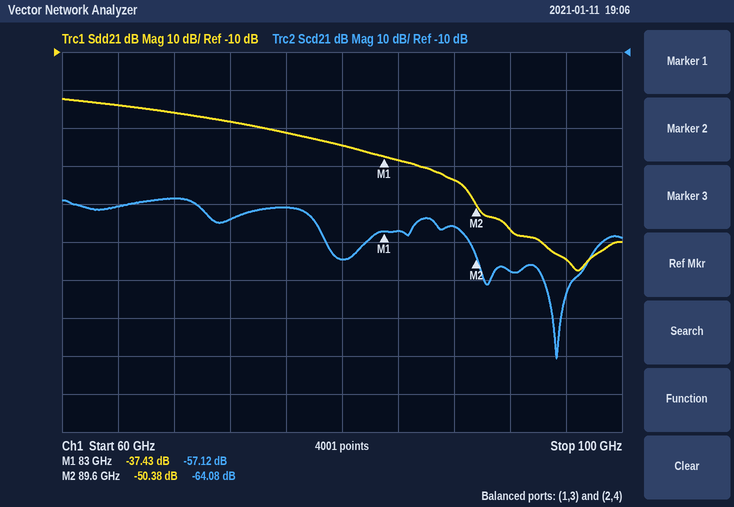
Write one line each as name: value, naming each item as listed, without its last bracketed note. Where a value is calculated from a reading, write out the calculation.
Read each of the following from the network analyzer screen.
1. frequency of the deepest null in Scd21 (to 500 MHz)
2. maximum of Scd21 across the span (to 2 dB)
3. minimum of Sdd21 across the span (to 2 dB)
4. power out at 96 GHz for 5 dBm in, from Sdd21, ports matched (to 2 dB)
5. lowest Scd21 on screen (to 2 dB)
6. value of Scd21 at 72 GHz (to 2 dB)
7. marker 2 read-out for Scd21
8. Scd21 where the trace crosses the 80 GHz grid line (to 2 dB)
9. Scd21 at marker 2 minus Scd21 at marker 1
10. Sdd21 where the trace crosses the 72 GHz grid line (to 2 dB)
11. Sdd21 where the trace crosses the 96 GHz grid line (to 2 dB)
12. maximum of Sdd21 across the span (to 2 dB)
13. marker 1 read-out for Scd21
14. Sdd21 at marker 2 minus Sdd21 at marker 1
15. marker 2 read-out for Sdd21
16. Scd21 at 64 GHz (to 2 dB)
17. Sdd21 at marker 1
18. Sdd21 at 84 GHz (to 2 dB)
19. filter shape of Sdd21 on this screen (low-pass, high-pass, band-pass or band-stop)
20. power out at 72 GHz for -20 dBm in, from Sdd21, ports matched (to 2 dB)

frequency of the deepest null in Scd21: 95.5 GHz
maximum of Scd21 across the span: -48 dB
minimum of Sdd21 across the span: -68 dB
power out at 96 GHz for 5 dBm in, from Sdd21, ports matched: 5 dBm + (-64 dB) = -60 dBm
lowest Scd21 on screen: -90 dB
value of Scd21 at 72 GHz: -54 dB
marker 2 read-out for Scd21: -64.08 dB
Scd21 where the trace crosses the 80 GHz grid line: -64 dB
Scd21 at marker 2 minus Scd21 at marker 1: -64.08 − (-57.12) = -6.96 dB
Sdd21 where the trace crosses the 72 GHz grid line: -28 dB
Sdd21 where the trace crosses the 96 GHz grid line: -64 dB
maximum of Sdd21 across the span: -22 dB
marker 1 read-out for Scd21: -57.12 dB
Sdd21 at marker 2 minus Sdd21 at marker 1: -50.38 − (-37.43) = -12.95 dB
marker 2 read-out for Sdd21: -50.38 dB
Scd21 at 64 GHz: -50 dB
Sdd21 at marker 1: -37.43 dB
Sdd21 at 84 GHz: -38 dB
filter shape of Sdd21 on this screen: low-pass
power out at 72 GHz for -20 dBm in, from Sdd21, ports matched: -20 dBm + (-28 dB) = -48 dBm
